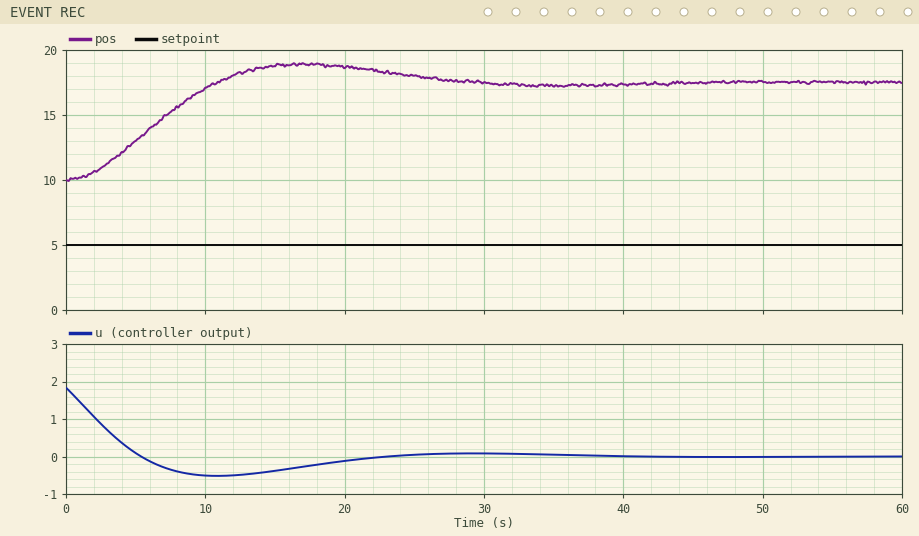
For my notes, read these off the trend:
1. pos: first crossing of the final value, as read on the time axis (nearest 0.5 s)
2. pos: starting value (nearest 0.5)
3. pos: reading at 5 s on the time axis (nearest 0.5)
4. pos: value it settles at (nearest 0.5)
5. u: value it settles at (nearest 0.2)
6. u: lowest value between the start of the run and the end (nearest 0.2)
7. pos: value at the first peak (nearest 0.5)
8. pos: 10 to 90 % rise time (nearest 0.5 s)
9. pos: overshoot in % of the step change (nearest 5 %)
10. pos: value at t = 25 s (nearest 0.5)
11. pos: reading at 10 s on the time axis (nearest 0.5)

11.0 s
10.0
13.0
17.5
0.0
-0.6
19.0
7.5 s
20 %
18.0
17.0
